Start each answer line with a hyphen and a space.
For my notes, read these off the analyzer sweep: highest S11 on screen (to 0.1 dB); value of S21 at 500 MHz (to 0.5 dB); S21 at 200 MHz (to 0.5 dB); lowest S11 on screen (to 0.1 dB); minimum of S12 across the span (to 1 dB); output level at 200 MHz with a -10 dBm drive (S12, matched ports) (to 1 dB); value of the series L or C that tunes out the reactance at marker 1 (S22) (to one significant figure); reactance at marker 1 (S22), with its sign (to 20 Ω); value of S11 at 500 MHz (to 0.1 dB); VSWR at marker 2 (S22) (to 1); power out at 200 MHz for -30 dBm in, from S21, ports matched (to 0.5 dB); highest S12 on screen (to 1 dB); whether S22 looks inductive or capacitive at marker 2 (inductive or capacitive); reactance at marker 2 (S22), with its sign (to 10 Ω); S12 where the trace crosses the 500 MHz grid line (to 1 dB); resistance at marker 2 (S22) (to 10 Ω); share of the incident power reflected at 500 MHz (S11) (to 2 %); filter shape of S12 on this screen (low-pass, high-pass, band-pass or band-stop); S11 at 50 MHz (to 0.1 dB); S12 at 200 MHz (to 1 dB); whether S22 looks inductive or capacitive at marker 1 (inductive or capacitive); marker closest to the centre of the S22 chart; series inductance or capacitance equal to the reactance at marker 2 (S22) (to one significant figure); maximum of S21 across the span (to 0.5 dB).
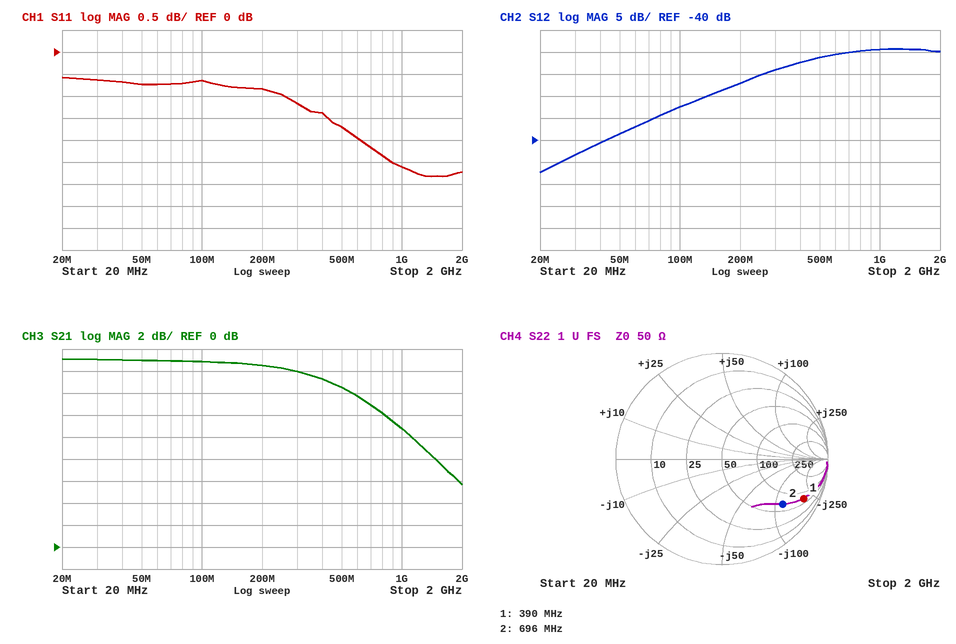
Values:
- -0.6 dB
- 14.5 dB
- 16.5 dB
- -2.8 dB
- -47 dB
- -37 dBm
- 80 nH
- -200 Ω
- -1.7 dB
- 6
- -13.5 dBm
- -19 dB
- capacitive
- -120 Ω
- -21 dB
- 70 Ω
- 68 %
- high-pass
- -0.7 dB
- -27 dB
- capacitive
- marker 2
- 2 pF
- 17.0 dB
